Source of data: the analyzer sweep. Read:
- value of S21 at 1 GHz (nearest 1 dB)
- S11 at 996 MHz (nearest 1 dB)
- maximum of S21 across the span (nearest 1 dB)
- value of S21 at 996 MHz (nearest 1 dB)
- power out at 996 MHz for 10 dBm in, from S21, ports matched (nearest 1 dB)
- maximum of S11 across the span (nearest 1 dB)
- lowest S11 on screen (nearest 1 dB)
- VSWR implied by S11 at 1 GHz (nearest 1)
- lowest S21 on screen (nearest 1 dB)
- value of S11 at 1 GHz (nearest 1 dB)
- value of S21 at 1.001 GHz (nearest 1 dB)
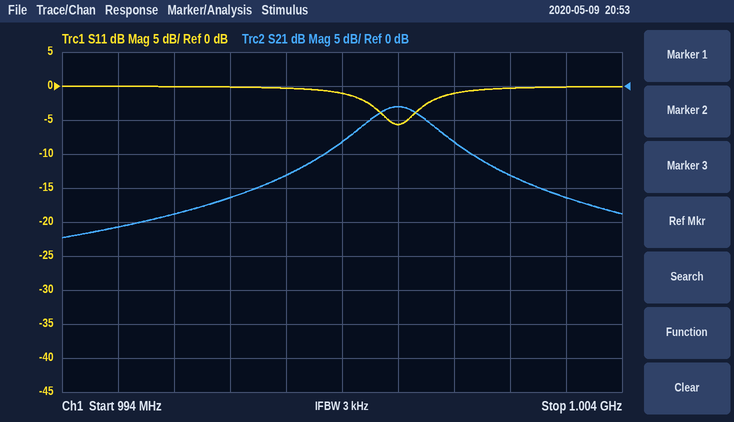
-3 dB
0 dB
-3 dB
-19 dB
-9 dBm
0 dB
-6 dB
3
-22 dB
-6 dB
-8 dB
